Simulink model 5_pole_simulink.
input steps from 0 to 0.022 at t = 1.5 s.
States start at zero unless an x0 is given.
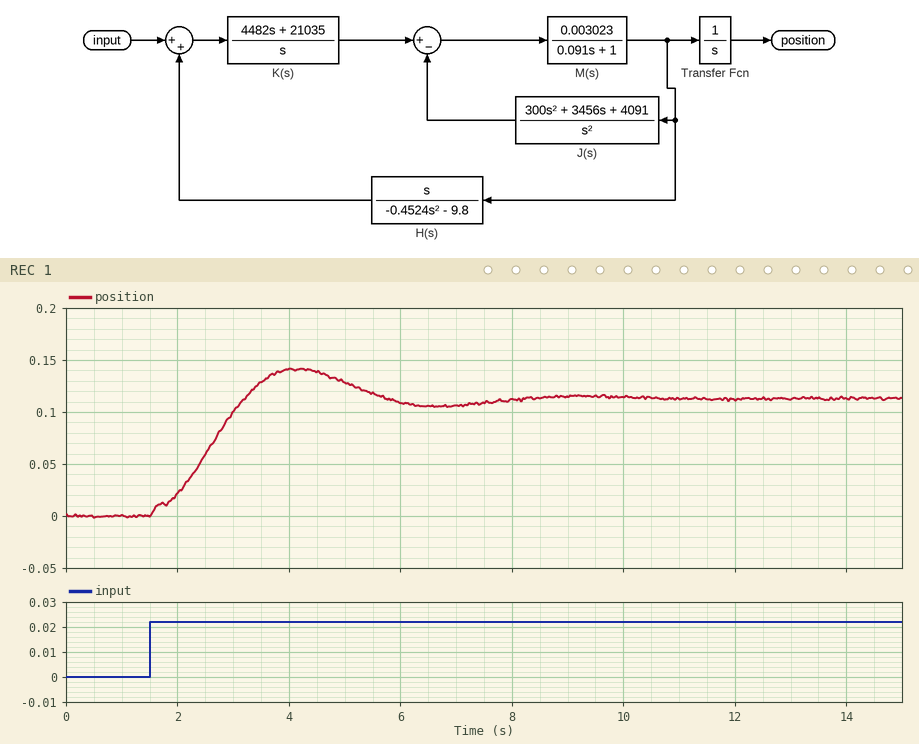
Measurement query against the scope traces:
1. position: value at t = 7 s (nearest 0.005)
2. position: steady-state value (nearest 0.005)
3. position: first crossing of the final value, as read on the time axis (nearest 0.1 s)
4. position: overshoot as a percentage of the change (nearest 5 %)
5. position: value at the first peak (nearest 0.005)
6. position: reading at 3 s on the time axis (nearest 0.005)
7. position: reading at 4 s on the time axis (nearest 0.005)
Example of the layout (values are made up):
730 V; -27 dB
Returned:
0.105; 0.115; 3.2 s; 25 %; 0.140; 0.100; 0.140
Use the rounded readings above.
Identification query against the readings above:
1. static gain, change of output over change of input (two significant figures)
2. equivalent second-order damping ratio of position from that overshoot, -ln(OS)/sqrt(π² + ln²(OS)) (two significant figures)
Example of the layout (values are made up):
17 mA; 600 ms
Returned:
5.2; 0.40
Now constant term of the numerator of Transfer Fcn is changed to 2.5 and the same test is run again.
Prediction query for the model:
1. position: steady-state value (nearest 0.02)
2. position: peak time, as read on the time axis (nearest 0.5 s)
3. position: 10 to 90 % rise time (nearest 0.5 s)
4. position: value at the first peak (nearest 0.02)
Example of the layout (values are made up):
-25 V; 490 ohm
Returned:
0.28; 4.0 s; 1.5 s; 0.36
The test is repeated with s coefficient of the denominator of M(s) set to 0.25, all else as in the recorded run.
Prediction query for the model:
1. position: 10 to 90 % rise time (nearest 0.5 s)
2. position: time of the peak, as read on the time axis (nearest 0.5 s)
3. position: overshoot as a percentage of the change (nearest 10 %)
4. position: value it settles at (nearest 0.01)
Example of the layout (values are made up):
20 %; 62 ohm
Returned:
1.5 s; 4.0 s; 30 %; 0.11
